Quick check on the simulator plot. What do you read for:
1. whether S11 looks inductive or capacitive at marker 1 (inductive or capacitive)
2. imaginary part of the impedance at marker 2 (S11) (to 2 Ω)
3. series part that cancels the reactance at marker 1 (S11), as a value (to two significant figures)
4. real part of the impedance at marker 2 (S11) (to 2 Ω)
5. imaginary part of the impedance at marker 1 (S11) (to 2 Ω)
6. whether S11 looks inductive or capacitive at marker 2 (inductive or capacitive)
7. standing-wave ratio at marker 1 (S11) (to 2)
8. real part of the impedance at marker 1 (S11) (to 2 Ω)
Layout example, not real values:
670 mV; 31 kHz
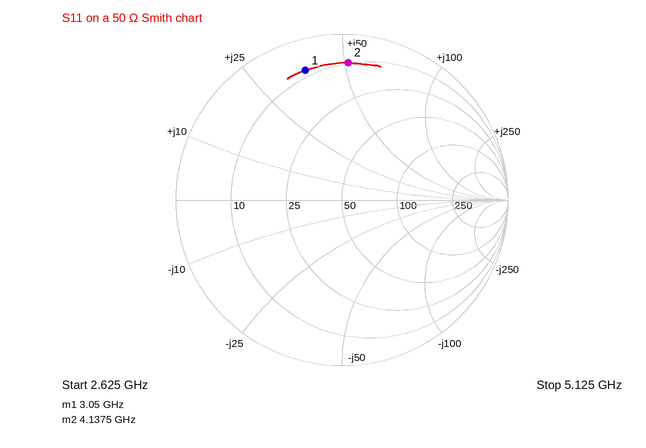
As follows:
inductive; +52 Ω; 1.4 pF; 10 Ω; +38 Ω; inductive; 10; 8 Ω
